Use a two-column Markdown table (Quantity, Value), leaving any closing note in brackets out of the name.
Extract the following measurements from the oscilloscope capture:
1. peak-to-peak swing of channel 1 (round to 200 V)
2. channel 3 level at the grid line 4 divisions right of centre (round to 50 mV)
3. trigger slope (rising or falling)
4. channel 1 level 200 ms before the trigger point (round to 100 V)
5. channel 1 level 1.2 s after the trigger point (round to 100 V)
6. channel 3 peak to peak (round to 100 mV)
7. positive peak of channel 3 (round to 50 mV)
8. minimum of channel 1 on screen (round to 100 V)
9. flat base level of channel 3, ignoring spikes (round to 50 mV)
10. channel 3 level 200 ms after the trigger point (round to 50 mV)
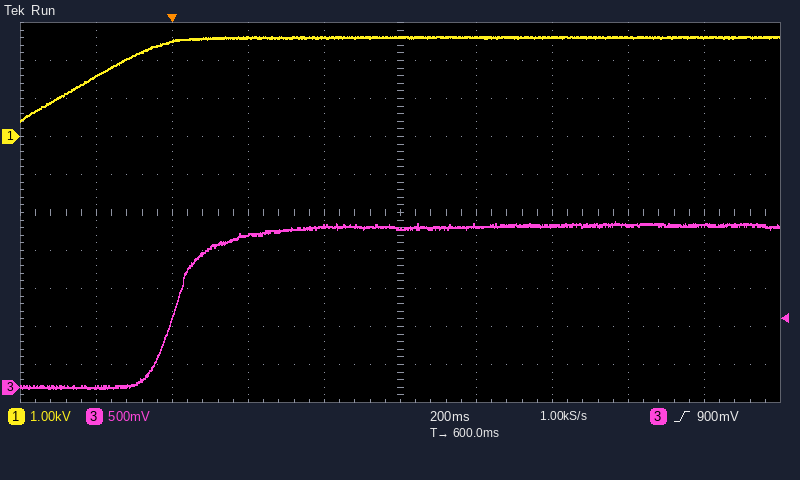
| Quantity | Value |
|---|---|
| peak-to-peak swing of channel 1 | 2.2 kV |
| channel 3 level at the grid line 4 divisions right of centre | 2.15 V |
| trigger slope | rising |
| channel 1 level 200 ms before the trigger point | 1.6 kV |
| channel 1 level 1.2 s after the trigger point | 2.6 kV |
| channel 3 peak to peak | 2.20 V |
| positive peak of channel 3 | 2.20 V |
| minimum of channel 1 on screen | 400 V |
| flat base level of channel 3, ignoring spikes | 0 mV |
| channel 3 level 200 ms after the trigger point | 2.00 V |
